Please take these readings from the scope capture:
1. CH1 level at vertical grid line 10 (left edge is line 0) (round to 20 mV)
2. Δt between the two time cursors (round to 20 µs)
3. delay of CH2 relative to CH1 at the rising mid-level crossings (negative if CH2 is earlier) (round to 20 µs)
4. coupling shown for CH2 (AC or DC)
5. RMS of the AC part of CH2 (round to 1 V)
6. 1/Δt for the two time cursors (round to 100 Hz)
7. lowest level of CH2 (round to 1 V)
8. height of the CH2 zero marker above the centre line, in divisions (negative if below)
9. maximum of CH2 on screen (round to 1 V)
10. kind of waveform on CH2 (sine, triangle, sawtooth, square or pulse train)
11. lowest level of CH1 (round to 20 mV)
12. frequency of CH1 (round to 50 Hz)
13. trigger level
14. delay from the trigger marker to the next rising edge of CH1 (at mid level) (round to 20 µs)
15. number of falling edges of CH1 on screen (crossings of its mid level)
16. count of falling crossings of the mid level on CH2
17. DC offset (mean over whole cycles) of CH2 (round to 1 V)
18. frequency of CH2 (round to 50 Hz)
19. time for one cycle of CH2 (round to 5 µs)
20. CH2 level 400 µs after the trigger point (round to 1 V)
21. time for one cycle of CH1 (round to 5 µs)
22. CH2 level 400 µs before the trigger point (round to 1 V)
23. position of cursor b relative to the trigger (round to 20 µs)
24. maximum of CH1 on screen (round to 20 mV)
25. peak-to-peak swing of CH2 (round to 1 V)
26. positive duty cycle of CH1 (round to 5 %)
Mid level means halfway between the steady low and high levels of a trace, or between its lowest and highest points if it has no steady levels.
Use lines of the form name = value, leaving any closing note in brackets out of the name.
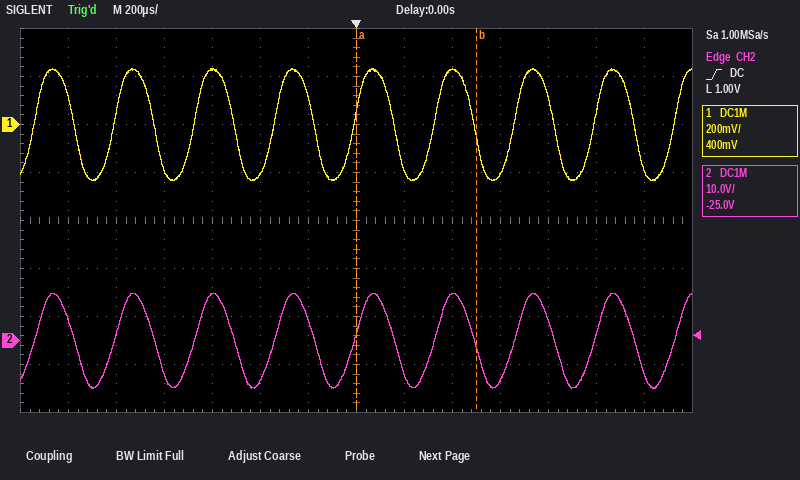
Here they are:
CH1 level at vertical grid line 10 (left edge is line 0) = -200 mV
Δt between the two time cursors = 500 µs
delay of CH2 relative to CH1 at the rising mid-level crossings (negative if CH2 is earlier) = 0 µs
coupling shown for CH2 = DC
RMS of the AC part of CH2 = 7 V
1/Δt for the two time cursors = 2.0 kHz
lowest level of CH2 = -10 V
height of the CH2 zero marker above the centre line, in divisions = -2.5 div
maximum of CH2 on screen = 10 V
kind of waveform on CH2 = sine
lowest level of CH1 = -240 mV
frequency of CH1 = 3.00 kHz
trigger level = 1.00 V
delay from the trigger marker to the next rising edge of CH1 (at mid level) = 320 µs
number of falling edges of CH1 on screen = 8
count of falling crossings of the mid level on CH2 = 8
DC offset (mean over whole cycles) of CH2 = 0 V
frequency of CH2 = 3.00 kHz
time for one cycle of CH2 = 335 µs
CH2 level 400 µs after the trigger point = 10 V
time for one cycle of CH1 = 335 µs
CH2 level 400 µs before the trigger point = -8 V
position of cursor b relative to the trigger = +500 µs
maximum of CH1 on screen = 240 mV
peak-to-peak swing of CH2 = 20 V
positive duty cycle of CH1 = 50 %
